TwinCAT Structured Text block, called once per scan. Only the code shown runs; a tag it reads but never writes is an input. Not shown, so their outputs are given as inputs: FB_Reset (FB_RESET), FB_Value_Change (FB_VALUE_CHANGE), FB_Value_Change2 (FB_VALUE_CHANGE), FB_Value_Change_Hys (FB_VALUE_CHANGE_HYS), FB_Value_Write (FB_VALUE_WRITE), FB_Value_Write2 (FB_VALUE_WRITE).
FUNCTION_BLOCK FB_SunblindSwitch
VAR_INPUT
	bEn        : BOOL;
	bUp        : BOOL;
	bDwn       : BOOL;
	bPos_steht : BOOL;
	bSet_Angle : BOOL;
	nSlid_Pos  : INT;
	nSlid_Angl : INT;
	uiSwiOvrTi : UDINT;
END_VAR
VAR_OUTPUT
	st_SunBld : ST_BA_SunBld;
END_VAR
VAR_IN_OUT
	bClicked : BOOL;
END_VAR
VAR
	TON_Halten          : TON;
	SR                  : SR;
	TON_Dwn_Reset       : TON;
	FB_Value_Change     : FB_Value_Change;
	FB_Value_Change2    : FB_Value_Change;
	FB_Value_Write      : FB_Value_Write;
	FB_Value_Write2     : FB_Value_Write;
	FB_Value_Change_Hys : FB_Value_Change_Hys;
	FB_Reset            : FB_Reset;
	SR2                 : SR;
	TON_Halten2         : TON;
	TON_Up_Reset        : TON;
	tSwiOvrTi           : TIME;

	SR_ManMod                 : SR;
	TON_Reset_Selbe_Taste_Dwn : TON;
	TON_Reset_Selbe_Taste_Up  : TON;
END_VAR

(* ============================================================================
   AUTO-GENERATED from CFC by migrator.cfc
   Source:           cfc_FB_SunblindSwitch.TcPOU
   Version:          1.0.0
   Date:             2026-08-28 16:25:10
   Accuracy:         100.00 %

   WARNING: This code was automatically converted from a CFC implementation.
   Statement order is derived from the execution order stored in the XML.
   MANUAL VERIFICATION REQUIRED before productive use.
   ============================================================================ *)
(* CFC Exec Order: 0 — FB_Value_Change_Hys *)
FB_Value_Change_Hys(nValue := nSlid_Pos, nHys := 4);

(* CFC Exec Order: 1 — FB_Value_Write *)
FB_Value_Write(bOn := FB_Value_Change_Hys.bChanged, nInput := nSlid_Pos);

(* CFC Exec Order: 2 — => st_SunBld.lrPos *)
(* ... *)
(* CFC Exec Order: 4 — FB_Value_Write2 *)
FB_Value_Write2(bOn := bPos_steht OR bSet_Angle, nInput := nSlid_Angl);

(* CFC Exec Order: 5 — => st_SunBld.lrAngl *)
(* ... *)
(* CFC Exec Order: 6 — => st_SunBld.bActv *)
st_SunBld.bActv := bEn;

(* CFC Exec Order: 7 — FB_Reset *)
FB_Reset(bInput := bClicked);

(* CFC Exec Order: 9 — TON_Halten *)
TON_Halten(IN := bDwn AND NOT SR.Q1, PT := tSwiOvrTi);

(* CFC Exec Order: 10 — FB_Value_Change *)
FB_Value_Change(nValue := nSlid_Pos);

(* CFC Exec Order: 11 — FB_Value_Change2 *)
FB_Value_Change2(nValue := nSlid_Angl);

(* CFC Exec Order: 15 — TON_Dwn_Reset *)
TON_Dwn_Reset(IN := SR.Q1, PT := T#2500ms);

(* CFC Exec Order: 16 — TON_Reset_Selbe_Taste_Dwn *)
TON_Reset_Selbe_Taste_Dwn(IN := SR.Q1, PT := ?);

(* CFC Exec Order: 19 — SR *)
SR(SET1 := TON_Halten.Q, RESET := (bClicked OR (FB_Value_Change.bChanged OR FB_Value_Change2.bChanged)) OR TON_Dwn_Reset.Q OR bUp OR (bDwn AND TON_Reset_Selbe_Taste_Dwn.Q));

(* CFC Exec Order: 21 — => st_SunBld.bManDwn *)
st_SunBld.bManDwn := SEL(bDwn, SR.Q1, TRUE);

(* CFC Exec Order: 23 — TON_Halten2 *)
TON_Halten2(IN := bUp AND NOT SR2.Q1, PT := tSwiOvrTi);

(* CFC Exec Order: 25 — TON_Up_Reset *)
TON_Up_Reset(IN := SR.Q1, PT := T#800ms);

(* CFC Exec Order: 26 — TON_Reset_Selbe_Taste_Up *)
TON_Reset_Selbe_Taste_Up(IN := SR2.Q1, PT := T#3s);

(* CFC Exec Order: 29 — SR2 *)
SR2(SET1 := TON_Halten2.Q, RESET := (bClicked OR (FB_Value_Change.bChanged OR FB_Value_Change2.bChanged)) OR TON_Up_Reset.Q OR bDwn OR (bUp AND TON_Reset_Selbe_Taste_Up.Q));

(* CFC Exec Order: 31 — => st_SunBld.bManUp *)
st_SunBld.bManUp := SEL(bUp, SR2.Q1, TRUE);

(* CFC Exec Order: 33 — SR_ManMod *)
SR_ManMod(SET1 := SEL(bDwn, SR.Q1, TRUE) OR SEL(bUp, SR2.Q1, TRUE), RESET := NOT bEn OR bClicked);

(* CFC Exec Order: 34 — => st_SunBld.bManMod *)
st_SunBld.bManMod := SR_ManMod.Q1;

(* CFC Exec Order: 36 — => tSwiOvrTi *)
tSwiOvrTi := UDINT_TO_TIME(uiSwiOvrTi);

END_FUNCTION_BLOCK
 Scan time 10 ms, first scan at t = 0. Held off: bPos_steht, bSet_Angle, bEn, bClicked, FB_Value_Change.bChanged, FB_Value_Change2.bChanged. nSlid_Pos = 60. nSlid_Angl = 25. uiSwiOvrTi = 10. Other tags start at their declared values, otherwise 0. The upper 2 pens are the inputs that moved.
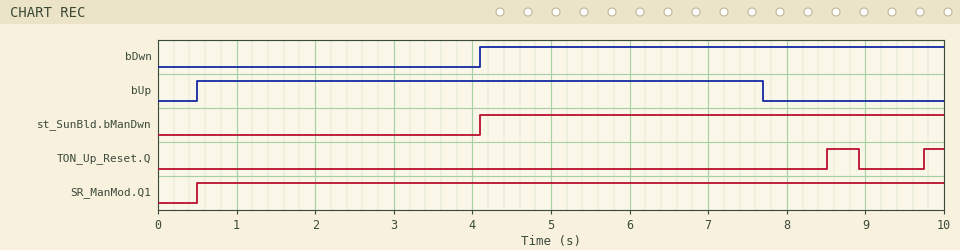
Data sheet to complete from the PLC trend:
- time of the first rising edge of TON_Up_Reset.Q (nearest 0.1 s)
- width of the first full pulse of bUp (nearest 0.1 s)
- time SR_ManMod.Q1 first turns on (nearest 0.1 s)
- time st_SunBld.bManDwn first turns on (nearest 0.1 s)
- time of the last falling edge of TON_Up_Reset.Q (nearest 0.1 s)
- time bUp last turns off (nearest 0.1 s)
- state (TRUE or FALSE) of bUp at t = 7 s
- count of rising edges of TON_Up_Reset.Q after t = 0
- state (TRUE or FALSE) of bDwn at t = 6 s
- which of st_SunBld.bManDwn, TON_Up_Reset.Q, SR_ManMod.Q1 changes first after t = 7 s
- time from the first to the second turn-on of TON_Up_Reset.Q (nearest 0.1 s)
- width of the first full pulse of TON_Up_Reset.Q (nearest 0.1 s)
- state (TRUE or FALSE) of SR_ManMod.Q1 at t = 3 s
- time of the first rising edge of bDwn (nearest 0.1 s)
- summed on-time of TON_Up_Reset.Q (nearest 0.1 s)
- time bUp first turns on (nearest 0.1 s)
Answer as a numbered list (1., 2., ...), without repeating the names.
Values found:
1. 8.5 s
2. 7.2 s
3. 0.5 s
4. 4.1 s
5. 8.9 s
6. 7.7 s
7. TRUE
8. 2
9. TRUE
10. TON_Up_Reset.Q
11. 1.2 s
12. 0.4 s
13. TRUE
14. 4.1 s
15. 0.7 s
16. 0.5 s
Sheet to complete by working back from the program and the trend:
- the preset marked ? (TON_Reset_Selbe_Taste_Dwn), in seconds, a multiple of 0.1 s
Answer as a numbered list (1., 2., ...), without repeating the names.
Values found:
1. 1.2 s
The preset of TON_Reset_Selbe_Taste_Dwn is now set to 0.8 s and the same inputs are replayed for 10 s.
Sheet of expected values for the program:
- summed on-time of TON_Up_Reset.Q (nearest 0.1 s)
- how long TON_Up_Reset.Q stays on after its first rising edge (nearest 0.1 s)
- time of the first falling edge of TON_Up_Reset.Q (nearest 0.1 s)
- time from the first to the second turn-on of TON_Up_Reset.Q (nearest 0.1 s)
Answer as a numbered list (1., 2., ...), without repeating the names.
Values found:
1. 0.0 s
2. 0.0 s
3. 8.5 s
4. 0.8 s
